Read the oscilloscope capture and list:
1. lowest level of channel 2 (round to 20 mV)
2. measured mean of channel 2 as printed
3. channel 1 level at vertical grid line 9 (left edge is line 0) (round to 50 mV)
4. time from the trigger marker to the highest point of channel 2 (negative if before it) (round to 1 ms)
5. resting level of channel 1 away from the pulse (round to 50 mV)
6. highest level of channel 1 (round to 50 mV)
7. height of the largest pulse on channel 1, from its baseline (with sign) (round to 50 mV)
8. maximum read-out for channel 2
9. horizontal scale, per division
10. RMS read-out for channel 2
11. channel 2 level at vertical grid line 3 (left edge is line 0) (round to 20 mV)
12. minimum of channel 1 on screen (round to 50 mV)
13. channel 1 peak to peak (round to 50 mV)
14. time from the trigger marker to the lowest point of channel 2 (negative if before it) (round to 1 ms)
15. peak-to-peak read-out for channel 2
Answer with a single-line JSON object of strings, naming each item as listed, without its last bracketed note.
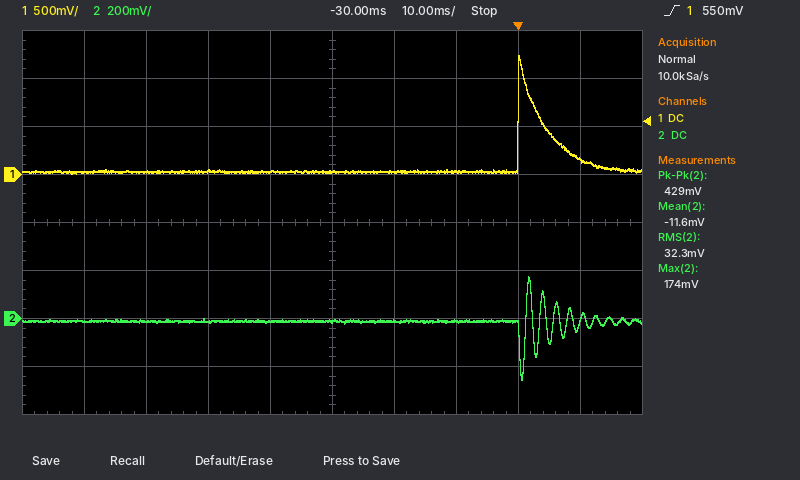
{"lowest level of channel 2": "-260 mV", "measured mean of channel 2 as printed": "-11.6 mV", "channel 1 level at vertical grid line 9 (left edge is line 0)": "150 mV", "time from the trigger marker to the highest point of channel 2 (negative if before it)": "+2 ms", "resting level of channel 1 away from the pulse": "50 mV", "highest level of channel 1": "1.25 V", "height of the largest pulse on channel 1, from its baseline (with sign)": "+1.20 V", "maximum read-out for channel 2": "174 mV", "horizontal scale, per division": "10 ms", "RMS read-out for channel 2": "32.3 mV", "channel 2 level at vertical grid line 3 (left edge is line 0)": "-20 mV", "minimum of channel 1 on screen": "0 mV", "channel 1 peak to peak": "1.25 V", "time from the trigger marker to the lowest point of channel 2 (negative if before it)": "+1 ms", "peak-to-peak read-out for channel 2": "429 mV"}
